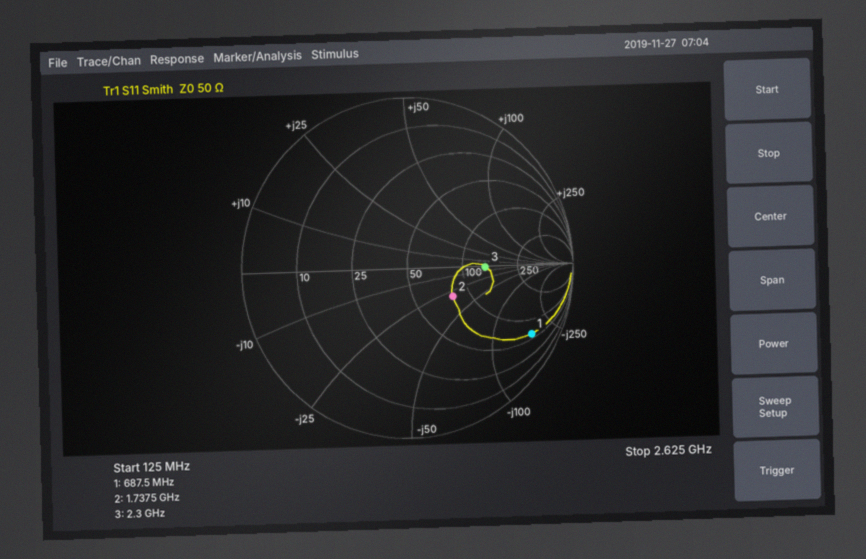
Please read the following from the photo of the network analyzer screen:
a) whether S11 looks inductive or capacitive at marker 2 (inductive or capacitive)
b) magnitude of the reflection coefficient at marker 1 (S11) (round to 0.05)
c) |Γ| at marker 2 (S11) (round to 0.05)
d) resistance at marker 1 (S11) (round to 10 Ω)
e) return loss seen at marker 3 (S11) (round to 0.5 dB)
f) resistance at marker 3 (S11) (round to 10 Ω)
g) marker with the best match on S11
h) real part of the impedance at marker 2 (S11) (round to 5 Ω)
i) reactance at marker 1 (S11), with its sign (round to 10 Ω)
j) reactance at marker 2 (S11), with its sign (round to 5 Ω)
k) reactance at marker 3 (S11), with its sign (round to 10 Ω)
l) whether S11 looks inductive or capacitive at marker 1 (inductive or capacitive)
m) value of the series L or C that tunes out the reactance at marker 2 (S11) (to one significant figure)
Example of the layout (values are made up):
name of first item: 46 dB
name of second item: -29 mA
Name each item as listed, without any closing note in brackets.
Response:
whether S11 looks inductive or capacitive at marker 2: capacitive
magnitude of the reflection coefficient at marker 1 (S11): 0.85
|Γ| at marker 2 (S11): 0.30
resistance at marker 1 (S11): 60 Ω
return loss seen at marker 3 (S11): 6.5 dB
resistance at marker 3 (S11): 140 Ω
marker with the best match on S11: marker 2
real part of the impedance at marker 2 (S11): 80 Ω
reactance at marker 1 (S11), with its sign: -170 Ω
reactance at marker 2 (S11), with its sign: -30 Ω
reactance at marker 3 (S11), with its sign: 0 Ω
whether S11 looks inductive or capacitive at marker 1: capacitive
value of the series L or C that tunes out the reactance at marker 2 (S11): 3 nH
